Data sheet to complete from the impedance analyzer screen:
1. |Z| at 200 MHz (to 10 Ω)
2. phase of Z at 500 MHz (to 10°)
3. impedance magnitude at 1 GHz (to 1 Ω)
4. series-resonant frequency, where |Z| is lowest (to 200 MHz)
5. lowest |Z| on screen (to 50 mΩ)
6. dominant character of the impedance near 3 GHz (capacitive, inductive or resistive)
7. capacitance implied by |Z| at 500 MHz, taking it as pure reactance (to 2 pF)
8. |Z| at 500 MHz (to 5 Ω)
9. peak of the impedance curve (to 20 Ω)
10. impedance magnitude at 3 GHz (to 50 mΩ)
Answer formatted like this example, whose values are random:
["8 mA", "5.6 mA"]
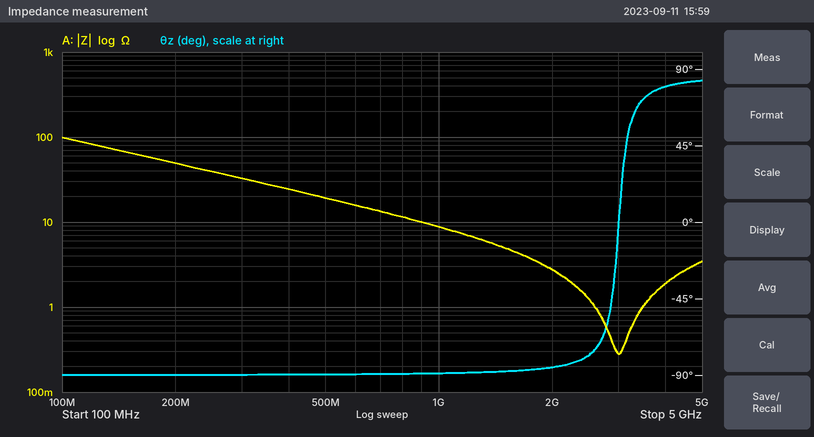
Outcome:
["50 Ω", "-90°", "9 Ω", "3.0 GHz", "300 mΩ", "resistive", "16 pF", "20 Ω", "100 Ω", "300 mΩ"]
